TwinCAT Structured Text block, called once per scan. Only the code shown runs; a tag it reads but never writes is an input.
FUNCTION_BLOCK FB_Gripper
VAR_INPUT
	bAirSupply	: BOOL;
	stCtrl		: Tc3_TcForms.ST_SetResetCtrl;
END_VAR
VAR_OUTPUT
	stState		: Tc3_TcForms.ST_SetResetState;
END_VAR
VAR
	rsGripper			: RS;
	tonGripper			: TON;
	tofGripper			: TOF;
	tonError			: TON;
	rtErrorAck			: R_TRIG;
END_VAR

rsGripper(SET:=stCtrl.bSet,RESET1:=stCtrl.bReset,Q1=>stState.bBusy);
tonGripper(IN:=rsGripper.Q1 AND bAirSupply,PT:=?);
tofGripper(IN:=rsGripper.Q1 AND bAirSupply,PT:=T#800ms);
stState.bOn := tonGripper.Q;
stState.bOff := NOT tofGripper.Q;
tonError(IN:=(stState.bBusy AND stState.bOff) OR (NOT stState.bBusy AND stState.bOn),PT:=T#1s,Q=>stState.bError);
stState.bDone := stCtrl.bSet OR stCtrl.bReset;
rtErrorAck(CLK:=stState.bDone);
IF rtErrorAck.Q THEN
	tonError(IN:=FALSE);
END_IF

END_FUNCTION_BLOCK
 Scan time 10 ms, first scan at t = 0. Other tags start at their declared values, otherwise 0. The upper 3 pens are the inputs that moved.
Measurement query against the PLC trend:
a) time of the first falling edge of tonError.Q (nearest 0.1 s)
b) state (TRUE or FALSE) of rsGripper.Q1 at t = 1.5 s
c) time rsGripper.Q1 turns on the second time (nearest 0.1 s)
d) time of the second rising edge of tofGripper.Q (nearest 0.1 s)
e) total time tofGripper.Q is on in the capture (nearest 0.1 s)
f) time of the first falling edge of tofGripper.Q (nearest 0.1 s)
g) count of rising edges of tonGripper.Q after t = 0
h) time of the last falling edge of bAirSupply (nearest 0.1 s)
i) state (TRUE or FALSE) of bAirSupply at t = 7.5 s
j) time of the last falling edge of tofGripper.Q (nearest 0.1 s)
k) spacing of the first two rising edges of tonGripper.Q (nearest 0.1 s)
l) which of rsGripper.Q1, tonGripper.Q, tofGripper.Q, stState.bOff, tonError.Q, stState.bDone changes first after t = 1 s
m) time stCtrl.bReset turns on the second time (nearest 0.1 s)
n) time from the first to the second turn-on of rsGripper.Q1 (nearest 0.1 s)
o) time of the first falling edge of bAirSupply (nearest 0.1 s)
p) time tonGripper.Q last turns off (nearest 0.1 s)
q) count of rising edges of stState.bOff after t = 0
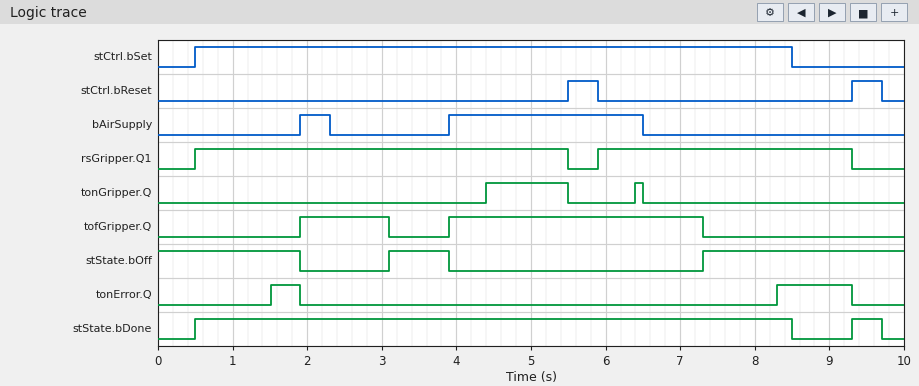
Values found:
1.9 s
TRUE
5.9 s
3.9 s
4.6 s
3.1 s
2
6.5 s
FALSE
7.3 s
2.0 s
tonError.Q
9.3 s
5.4 s
2.3 s
6.5 s
2
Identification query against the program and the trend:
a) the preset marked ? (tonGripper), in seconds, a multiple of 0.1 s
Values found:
0.5 s
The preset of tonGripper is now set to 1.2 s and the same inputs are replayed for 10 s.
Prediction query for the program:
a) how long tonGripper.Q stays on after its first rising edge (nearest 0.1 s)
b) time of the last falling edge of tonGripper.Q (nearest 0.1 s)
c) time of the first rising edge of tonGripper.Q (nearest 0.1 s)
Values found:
0.4 s
5.5 s
5.1 s
